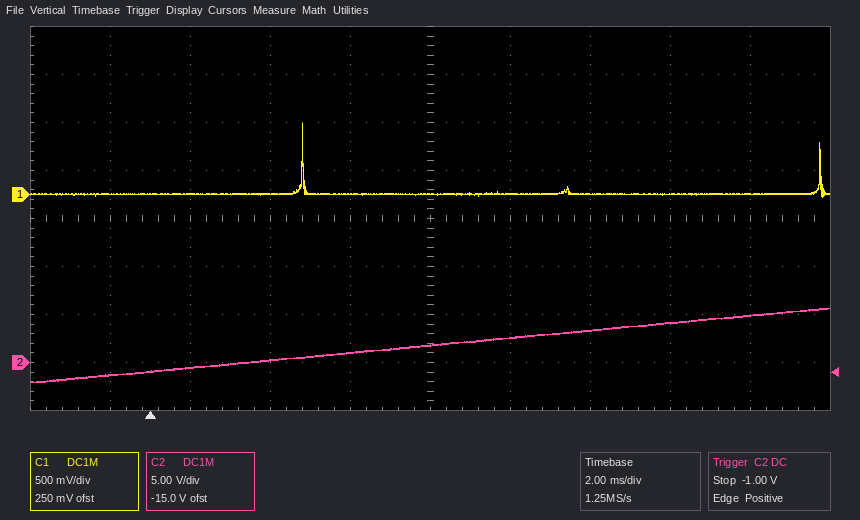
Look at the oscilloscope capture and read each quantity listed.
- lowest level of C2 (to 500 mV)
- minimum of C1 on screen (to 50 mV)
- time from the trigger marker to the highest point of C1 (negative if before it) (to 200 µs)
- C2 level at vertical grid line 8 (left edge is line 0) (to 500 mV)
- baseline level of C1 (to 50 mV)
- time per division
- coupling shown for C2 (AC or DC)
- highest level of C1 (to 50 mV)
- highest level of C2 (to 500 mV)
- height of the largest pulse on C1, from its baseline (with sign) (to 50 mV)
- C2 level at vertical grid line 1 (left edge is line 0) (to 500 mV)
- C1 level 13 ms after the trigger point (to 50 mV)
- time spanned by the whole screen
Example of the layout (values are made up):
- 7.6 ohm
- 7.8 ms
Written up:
- -2.0 V
- -50 mV
- +3.8 ms
- 4.0 V
- 0 mV
- 2 ms
- DC
- 750 mV
- 5.5 V
- +750 mV
- -1.5 V
- 0 mV
- 20 ms
